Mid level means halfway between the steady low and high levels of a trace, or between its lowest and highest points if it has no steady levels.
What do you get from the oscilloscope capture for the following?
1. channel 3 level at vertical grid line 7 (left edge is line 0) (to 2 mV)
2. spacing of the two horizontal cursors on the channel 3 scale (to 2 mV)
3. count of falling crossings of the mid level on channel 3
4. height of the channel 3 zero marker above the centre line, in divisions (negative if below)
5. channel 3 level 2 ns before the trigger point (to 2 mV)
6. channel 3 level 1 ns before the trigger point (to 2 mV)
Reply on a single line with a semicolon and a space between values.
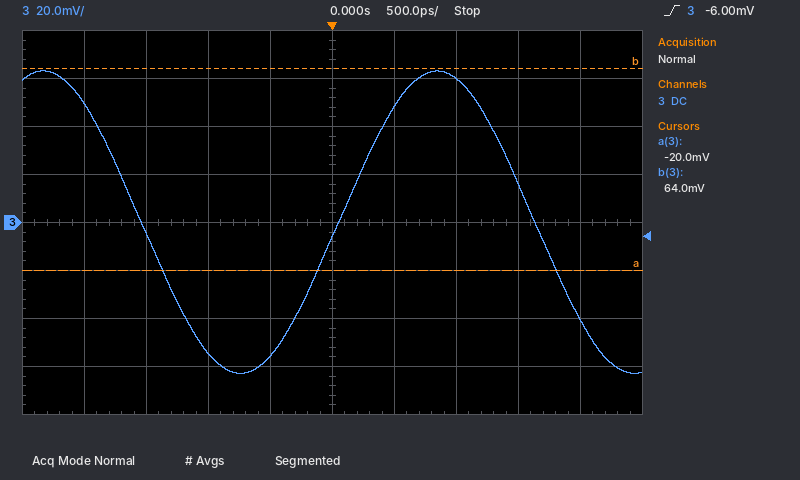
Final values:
60 mV; 84 mV; 2; 0.0 div; 50 mV; -54 mV
